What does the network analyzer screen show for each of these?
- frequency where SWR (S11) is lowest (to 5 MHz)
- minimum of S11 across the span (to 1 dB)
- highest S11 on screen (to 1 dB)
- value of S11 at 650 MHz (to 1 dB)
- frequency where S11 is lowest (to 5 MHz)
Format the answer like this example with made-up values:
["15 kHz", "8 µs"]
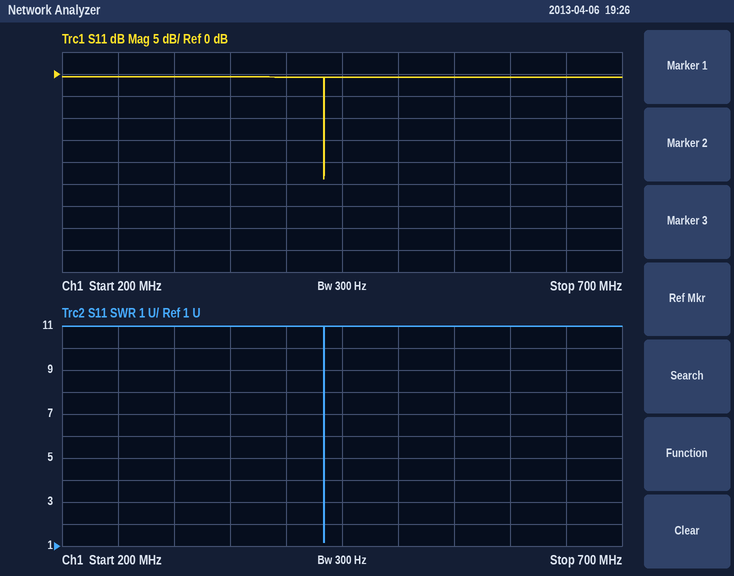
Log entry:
["435 MHz", "-24 dB", "-1 dB", "-1 dB", "435 MHz"]
